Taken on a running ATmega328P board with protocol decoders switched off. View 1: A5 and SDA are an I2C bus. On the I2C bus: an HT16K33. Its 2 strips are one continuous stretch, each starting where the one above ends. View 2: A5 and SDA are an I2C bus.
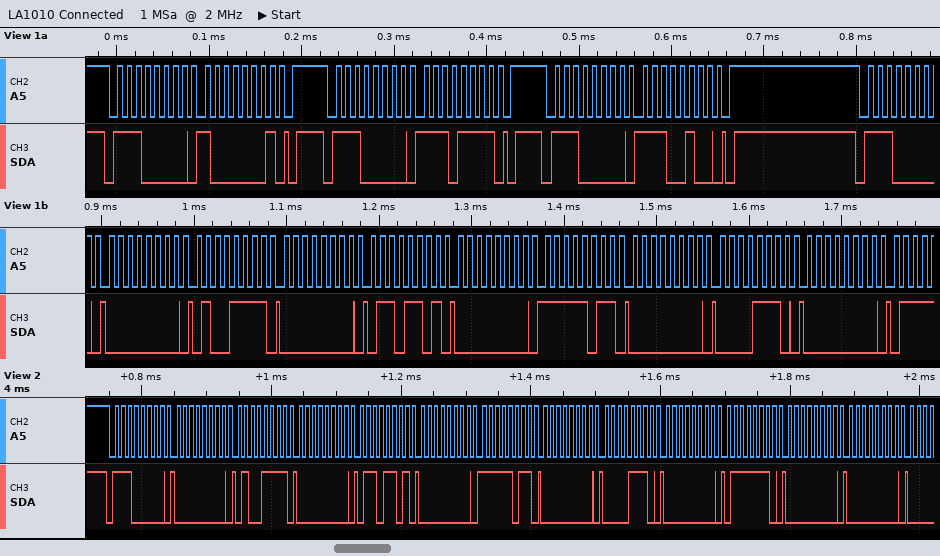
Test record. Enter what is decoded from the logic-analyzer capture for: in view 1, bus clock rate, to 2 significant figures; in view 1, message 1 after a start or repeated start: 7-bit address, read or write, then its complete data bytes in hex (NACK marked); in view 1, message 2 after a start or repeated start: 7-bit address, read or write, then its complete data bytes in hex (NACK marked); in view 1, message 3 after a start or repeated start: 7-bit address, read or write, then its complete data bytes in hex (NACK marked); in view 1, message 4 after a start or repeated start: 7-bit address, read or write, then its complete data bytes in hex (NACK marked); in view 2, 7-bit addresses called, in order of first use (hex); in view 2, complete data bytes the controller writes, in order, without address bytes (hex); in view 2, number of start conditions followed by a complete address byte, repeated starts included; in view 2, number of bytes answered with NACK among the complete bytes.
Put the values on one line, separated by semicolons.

100 kHz; 0x70 write: 81; 0x70 write: EF; 0x70 write: E4; 0x70 write: 00 4F 00 6D 00 FB 00 0E 00; 0x70; 00 4F 00 6D 00 FB 00 0E 00 7E 00 00; 1; 0
